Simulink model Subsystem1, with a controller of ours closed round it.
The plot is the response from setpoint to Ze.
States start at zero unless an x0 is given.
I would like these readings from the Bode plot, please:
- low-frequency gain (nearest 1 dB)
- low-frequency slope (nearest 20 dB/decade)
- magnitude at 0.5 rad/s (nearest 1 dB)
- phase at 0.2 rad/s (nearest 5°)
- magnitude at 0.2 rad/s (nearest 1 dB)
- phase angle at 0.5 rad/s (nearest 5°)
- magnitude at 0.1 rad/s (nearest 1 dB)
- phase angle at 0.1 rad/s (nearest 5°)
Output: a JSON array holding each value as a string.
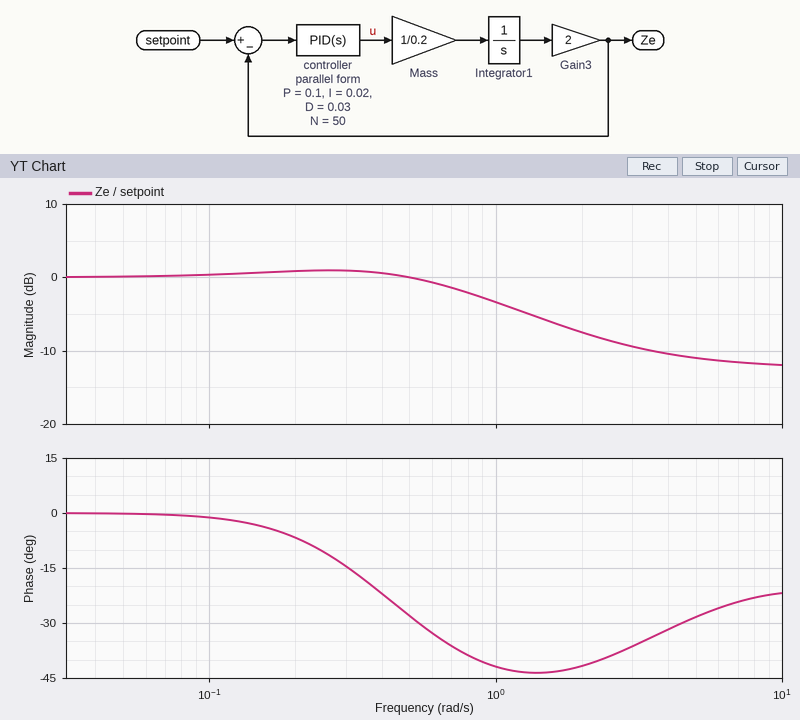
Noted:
["0 dB", "0 dB/decade", "0 dB", "-5°", "1 dB", "-30°", "0 dB", "0°"]
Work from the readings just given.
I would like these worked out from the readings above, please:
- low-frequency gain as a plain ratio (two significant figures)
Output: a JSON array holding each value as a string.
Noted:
["1.0"]
